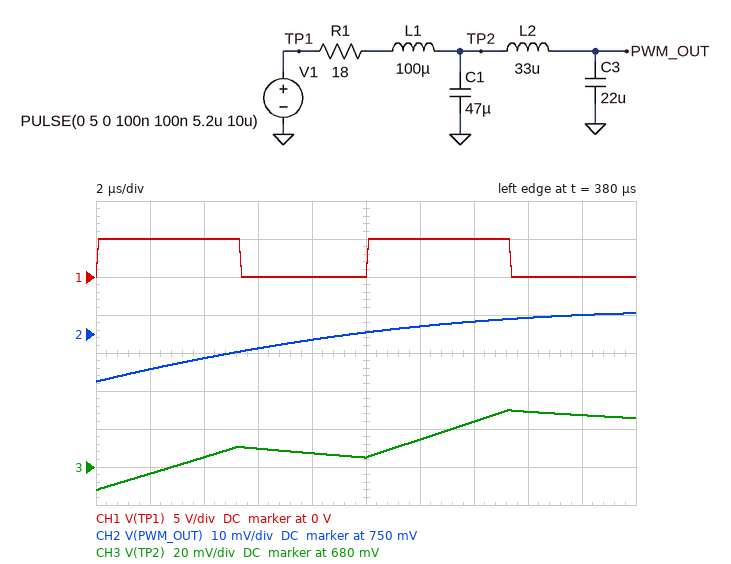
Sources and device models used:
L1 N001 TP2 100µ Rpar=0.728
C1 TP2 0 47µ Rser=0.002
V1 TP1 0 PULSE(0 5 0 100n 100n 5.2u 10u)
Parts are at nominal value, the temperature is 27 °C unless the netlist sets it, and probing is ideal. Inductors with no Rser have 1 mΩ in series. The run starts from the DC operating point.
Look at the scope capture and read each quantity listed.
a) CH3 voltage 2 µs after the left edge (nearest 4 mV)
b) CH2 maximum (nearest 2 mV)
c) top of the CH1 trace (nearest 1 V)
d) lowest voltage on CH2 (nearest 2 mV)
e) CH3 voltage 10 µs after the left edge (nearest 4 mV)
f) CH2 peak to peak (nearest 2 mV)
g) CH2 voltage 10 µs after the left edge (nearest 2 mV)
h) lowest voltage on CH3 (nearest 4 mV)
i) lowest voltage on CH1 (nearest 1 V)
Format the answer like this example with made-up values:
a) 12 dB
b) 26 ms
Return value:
a) 676 mV
b) 756 mV
c) 5 V
d) 738 mV
e) 684 mV
f) 18 mV
g) 750 mV
h) 668 mV
i) 0 V
